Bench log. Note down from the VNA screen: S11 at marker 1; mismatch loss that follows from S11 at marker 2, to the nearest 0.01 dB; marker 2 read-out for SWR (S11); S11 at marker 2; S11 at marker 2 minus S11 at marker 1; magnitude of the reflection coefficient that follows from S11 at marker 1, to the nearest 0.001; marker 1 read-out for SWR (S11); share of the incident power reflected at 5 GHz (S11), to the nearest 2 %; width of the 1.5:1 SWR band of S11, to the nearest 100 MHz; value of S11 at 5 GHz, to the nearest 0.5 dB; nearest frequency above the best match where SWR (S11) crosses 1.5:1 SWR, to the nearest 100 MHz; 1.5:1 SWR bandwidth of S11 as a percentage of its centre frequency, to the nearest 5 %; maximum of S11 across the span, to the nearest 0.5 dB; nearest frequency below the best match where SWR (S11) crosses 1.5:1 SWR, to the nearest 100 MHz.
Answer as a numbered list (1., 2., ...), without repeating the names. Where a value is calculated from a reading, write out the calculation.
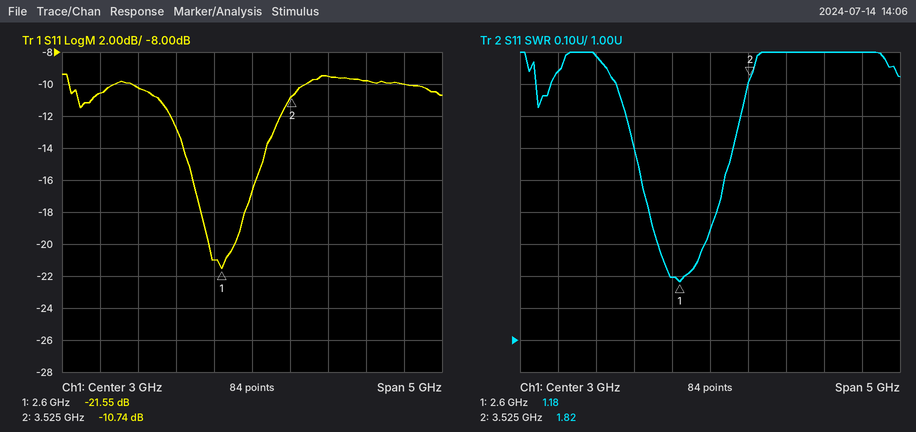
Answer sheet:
1. -21.55 dB
2. −10 log10(1 − 10^(-10.74/10)) ≈ 0.38 dB
3. 1.82
4. -10.74 dB
5. -10.74 − (-21.55) = 10.81 dB
6. 10^(-21.55/20) ≈ 0.084
7. 1.18
8. 10^(-10/10) ≈ 10 %
9. 3.2 GHz − 2.1 GHz = 1.1 GHz
10. -10.0 dB
11. 3.2 GHz
12. 1.1 GHz / 2.65 GHz ≈ 41.5 %, so 40 % to the nearest 5 %
13. -9.5 dB
14. 2.1 GHz
